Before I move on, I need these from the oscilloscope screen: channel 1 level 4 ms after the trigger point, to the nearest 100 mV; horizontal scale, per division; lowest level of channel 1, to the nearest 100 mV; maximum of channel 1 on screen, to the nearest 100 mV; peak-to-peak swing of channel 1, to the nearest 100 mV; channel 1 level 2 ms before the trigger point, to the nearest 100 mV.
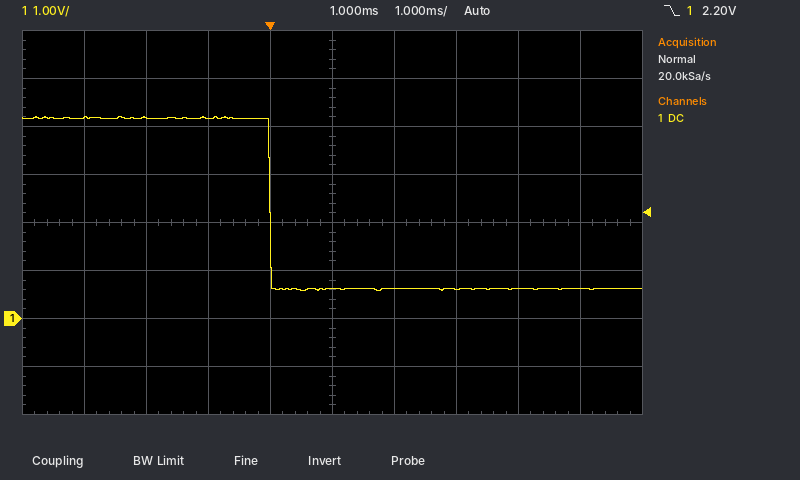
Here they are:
600 mV
1 ms
600 mV
4.2 V
3.6 V
4.2 V
